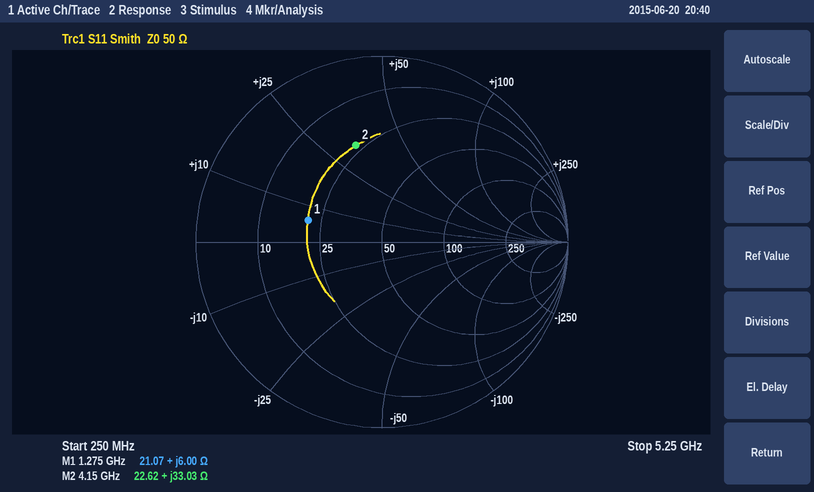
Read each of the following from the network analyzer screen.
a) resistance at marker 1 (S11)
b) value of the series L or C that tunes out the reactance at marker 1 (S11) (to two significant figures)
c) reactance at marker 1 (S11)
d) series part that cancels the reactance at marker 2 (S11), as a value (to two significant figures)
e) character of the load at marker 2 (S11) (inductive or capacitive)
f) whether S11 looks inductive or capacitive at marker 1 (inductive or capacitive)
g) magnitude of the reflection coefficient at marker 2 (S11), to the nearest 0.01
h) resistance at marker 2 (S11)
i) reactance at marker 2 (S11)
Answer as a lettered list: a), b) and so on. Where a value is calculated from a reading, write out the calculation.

a) 21.07 Ω
b) C = 1/(2π × 1.275 GHz × 6 Ω) ≈ 21 pF
c) +6.00 Ω
d) C = 1/(2π × 4.15 GHz × 33.03 Ω) ≈ 1.2 pF
e) inductive
f) inductive
g) 0.54
h) 22.62 Ω
i) +33.03 Ω
